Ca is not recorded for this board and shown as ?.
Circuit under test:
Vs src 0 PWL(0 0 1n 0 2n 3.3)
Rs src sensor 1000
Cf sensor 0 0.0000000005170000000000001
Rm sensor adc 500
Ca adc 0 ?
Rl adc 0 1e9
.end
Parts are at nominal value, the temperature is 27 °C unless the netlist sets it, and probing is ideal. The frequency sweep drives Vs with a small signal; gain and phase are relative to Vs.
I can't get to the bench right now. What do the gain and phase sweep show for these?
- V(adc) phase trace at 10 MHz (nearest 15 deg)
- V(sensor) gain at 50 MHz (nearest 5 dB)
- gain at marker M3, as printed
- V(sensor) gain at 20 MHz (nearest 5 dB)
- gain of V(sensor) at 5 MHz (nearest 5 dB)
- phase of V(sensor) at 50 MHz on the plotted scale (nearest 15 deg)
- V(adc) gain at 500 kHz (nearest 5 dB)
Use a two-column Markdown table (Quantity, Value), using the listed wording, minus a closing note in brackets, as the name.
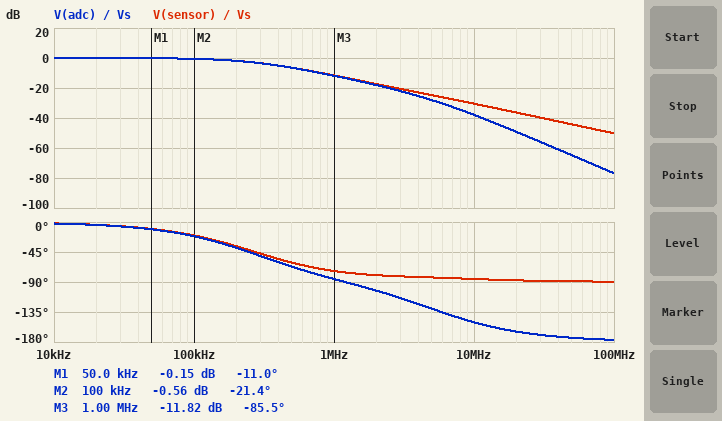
| Quantity | Value |
|---|---|
| V(adc) phase trace at 10 MHz | -150 deg |
| V(sensor) gain at 50 MHz | -45 dB |
| gain at marker M3, as printed | -11.82 dB |
| V(sensor) gain at 20 MHz | -35 dB |
| gain of V(sensor) at 5 MHz | -25 dB |
| phase of V(sensor) at 50 MHz on the plotted scale | -90 deg |
| V(adc) gain at 500 kHz | -5 dB |
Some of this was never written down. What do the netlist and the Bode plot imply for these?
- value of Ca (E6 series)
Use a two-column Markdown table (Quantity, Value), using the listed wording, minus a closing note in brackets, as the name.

| Quantity | Value |
|---|---|
| value of Ca | 68 pF |
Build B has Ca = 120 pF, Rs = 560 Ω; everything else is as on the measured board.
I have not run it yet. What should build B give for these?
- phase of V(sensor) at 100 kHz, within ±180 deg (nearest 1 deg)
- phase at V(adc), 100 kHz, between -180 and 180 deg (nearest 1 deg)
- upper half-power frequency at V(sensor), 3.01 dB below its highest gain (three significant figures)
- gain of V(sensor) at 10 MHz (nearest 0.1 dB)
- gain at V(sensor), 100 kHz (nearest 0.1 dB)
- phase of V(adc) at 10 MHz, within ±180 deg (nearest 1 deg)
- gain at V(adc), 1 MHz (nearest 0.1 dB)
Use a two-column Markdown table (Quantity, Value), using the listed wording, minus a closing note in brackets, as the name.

| Quantity | Value |
|---|---|
| phase of V(sensor) at 100 kHz, within ±180 deg | -13 deg |
| phase at V(adc), 100 kHz, between -180 and 180 deg | -15 deg |
| upper half-power frequency at V(sensor), 3.01 dB below its highest gain | 435 kHz |
| gain of V(sensor) at 10 MHz | -25.4 dB |
| gain at V(sensor), 100 kHz | -0.2 dB |
| phase of V(adc) at 10 MHz, within ±180 deg | -159 deg |
| gain at V(adc), 1 MHz | -8.4 dB |
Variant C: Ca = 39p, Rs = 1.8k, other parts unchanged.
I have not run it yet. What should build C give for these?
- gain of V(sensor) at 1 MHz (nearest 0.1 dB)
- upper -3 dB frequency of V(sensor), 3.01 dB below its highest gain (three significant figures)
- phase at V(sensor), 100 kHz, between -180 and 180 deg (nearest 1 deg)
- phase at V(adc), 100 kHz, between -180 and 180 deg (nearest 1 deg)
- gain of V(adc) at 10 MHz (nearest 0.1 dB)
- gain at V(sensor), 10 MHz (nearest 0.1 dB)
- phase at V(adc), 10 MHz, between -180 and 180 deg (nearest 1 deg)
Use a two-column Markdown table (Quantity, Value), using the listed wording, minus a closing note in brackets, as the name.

| Quantity | Value |
|---|---|
| gain of V(sensor) at 1 MHz | -16.1 dB |
| upper -3 dB frequency of V(sensor), 3.01 dB below its highest gain | 159 kHz |
| phase at V(sensor), 100 kHz, between -180 and 180 deg | -32 deg |
| phase at V(adc), 100 kHz, between -180 and 180 deg | -33 deg |
| gain of V(adc) at 10 MHz | -39.6 dB |
| gain at V(sensor), 10 MHz | -35.6 dB |
| phase at V(adc), 10 MHz, between -180 and 180 deg | -138 deg |
